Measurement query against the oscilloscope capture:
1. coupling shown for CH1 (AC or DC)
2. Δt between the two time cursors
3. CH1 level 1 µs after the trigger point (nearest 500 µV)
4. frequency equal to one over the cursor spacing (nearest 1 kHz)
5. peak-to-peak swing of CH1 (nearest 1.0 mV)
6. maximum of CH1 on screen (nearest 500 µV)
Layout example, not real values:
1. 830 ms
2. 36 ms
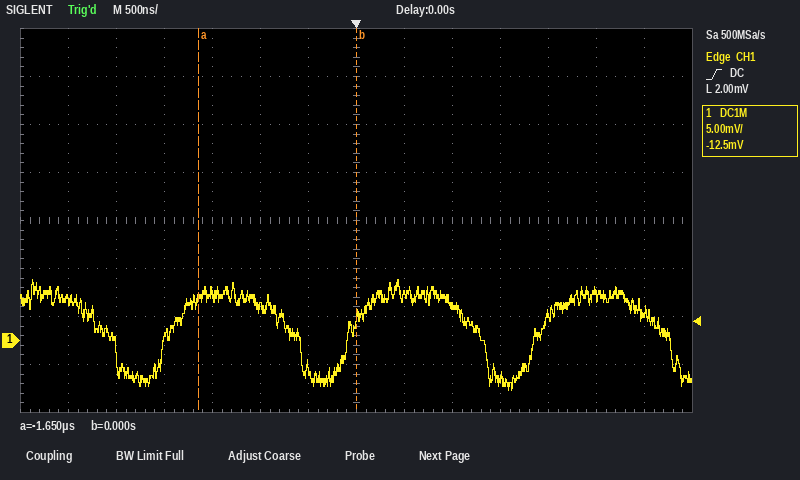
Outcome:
1. DC
2. 1.65 µs
3. 3.5 mV
4. 606 kHz
5. 12.0 mV
6. 6.5 mV
